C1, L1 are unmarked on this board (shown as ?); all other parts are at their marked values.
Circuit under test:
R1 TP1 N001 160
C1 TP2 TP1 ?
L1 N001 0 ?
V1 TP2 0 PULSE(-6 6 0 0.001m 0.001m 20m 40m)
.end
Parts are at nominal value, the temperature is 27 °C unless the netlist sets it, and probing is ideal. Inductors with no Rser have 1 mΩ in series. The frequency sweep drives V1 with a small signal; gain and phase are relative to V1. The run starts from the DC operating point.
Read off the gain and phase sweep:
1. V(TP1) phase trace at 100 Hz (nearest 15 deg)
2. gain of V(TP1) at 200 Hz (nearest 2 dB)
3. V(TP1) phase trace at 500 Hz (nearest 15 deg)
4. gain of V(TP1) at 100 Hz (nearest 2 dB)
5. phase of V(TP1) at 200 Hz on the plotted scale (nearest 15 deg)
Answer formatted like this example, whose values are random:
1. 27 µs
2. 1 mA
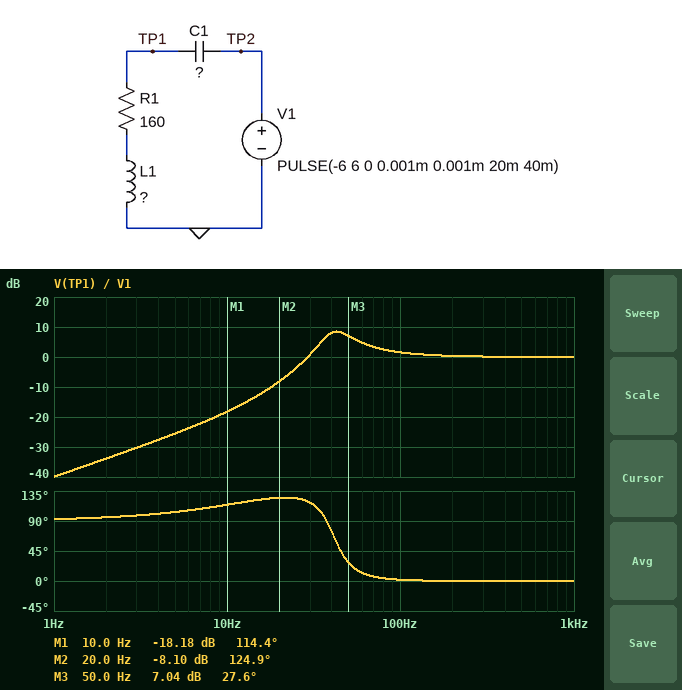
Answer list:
1. 0 deg
2. 0 dB
3. 0 deg
4. 2 dB
5. 0 deg
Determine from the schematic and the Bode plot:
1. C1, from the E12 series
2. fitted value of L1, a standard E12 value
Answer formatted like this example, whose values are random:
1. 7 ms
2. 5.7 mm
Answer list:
1. 10 µF
2. 1.5 H
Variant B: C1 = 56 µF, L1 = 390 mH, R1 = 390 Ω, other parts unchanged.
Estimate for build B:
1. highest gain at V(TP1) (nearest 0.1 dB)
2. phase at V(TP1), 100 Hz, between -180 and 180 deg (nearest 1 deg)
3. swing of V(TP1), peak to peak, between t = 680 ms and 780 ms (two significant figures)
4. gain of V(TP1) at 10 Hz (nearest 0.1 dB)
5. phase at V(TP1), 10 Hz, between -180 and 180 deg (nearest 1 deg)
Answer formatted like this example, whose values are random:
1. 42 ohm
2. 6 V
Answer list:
1. 0.3 dB
2. 3 deg
3. 17 V
4. -1.6 dB
5. 37 deg
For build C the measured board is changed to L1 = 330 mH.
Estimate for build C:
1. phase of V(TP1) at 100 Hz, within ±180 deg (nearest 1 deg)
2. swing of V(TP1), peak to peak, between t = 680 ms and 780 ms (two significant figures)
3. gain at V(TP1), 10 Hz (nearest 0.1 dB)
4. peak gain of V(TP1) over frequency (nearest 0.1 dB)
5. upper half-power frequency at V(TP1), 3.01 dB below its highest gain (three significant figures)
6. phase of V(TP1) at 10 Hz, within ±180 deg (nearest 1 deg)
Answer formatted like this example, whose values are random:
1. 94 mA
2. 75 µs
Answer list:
1. 36 deg
2. 24 V
3. -19.8 dB
4. 3.9 dB
5. 269 Hz
6. 92 deg
